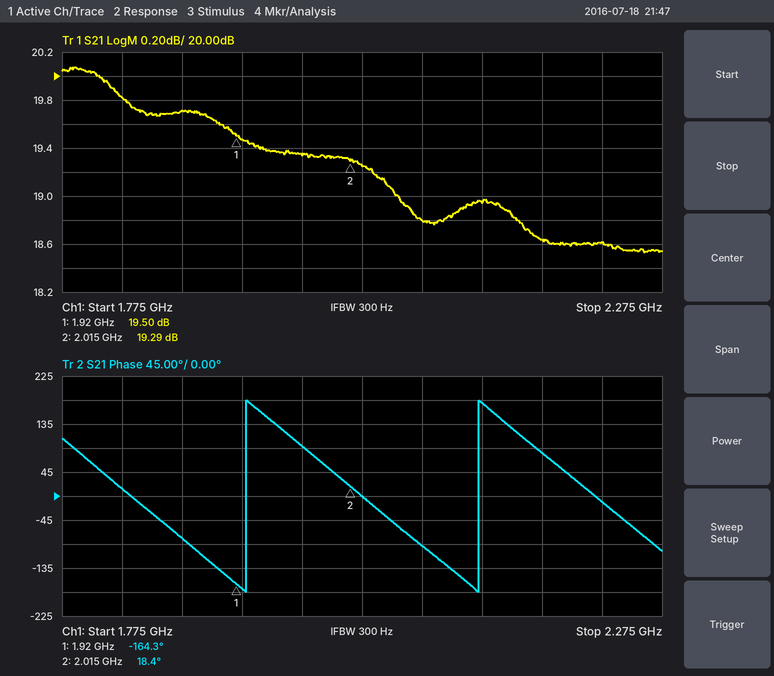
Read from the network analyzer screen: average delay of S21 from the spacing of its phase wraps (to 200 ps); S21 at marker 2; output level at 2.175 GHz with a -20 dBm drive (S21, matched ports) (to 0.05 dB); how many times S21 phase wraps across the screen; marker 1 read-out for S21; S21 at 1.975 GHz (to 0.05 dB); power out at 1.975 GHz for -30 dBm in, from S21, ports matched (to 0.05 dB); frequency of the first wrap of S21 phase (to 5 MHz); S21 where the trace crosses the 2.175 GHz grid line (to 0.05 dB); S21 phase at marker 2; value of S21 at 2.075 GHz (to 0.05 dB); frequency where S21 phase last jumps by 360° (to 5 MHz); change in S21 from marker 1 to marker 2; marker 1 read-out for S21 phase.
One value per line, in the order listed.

5.2 ns
19.29 dB
-1.35 dBm
2
19.50 dB
19.35 dB
-10.65 dBm
1.930 GHz
18.65 dB
18.4°
18.80 dB
2.120 GHz
-0.21 dB
-164.3°
